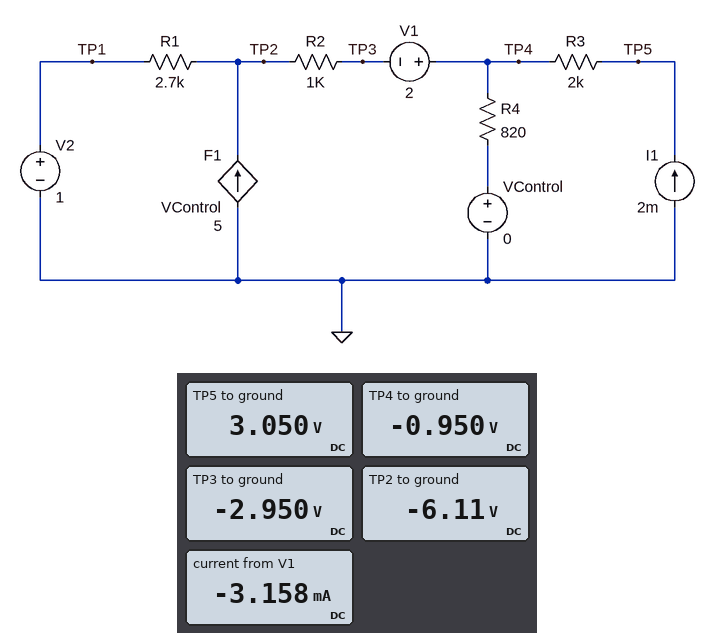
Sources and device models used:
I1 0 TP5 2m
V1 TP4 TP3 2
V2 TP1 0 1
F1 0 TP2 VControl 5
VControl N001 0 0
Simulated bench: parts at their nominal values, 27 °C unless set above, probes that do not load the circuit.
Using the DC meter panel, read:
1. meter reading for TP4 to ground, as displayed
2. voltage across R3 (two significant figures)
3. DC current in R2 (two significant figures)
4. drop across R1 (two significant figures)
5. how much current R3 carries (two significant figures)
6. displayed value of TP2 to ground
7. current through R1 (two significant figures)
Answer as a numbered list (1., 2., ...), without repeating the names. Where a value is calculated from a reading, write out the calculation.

1. -0.950 V
2. 3.05 V - (-950 mV) = 4.0 V
3. (-2.95 V - (-6.11 V)) / 1 kΩ = 3.2 mA
4. 1 V - (-6.11 V) = 7.1 V
5. (3.05 V - (-950 mV)) / 2 kΩ = 2.0 mA
6. -6.11 V
7. (1 V - (-6.11 V)) / 2.7 kΩ = 2.6 mA
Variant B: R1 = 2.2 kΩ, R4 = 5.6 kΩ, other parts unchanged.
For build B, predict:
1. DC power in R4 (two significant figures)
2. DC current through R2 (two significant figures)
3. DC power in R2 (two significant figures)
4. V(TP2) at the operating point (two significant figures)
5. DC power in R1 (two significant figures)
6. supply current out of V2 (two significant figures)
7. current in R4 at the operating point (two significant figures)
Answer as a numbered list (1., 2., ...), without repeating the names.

1. 100 mW
2. 6.3 mA
3. 39 mW
4. -32 V
5. 500 mW
6. 15 mA
7. 4.3 mA
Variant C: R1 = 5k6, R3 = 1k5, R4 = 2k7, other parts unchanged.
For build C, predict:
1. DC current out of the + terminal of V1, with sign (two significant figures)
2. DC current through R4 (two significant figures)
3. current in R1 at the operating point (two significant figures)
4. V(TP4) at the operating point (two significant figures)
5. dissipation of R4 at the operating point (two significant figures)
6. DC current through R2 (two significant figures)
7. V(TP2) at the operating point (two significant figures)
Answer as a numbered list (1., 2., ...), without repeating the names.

1. -2.9 mA
2. 870 µA
3. 1.5 mA
4. -2.3 V
5. 2.0 mW
6. 2.9 mA
7. -7.2 V
